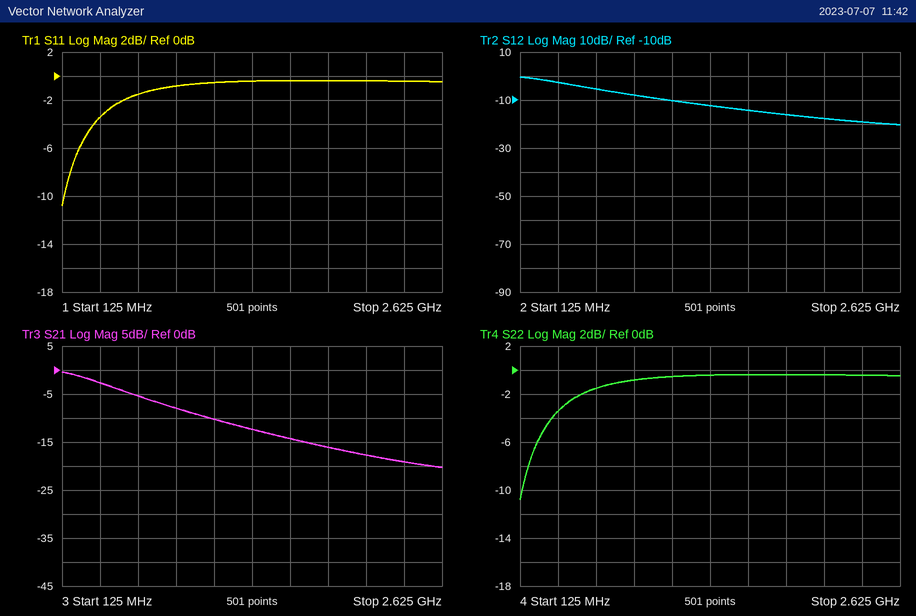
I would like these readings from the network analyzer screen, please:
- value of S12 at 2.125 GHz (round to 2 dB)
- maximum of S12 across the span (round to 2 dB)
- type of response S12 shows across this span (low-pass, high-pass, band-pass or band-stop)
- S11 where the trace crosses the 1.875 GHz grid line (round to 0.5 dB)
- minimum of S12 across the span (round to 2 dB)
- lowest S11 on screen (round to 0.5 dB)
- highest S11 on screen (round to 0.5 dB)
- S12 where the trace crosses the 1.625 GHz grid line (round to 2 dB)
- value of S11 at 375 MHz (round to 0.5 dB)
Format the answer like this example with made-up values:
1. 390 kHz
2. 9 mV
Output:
1. -18 dB
2. 0 dB
3. low-pass
4. -0.5 dB
5. -20 dB
6. -11.0 dB
7. -0.5 dB
8. -14 dB
9. -3.5 dB
